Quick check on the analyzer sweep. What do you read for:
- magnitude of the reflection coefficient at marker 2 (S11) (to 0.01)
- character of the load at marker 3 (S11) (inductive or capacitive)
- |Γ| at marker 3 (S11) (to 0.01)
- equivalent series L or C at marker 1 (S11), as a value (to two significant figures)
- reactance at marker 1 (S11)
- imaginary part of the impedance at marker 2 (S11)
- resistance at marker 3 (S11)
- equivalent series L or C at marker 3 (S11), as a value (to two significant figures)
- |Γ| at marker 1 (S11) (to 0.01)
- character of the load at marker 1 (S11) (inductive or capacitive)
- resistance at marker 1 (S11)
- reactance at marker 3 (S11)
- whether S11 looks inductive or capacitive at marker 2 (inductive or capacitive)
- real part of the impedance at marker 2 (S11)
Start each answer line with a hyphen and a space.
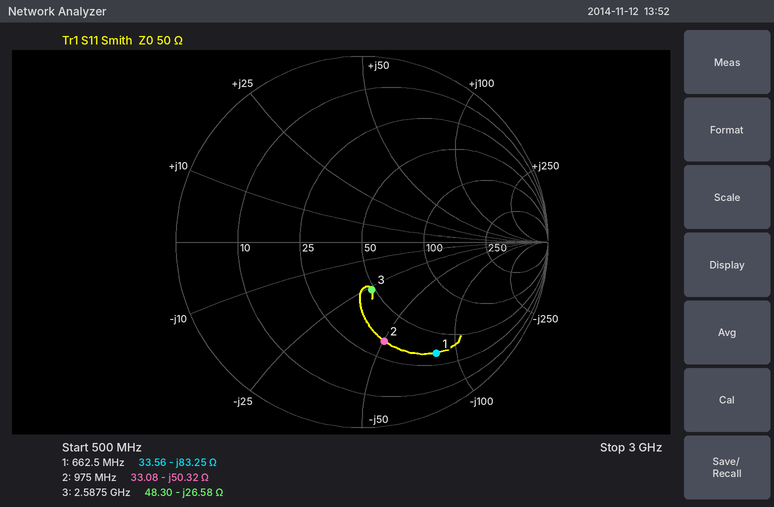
- 0.55
- capacitive
- 0.26
- 2.9 pF
- -83.25 Ω
- -50.32 Ω
- 48.30 Ω
- 2.3 pF
- 0.72
- capacitive
- 33.56 Ω
- -26.58 Ω
- capacitive
- 33.08 Ω
